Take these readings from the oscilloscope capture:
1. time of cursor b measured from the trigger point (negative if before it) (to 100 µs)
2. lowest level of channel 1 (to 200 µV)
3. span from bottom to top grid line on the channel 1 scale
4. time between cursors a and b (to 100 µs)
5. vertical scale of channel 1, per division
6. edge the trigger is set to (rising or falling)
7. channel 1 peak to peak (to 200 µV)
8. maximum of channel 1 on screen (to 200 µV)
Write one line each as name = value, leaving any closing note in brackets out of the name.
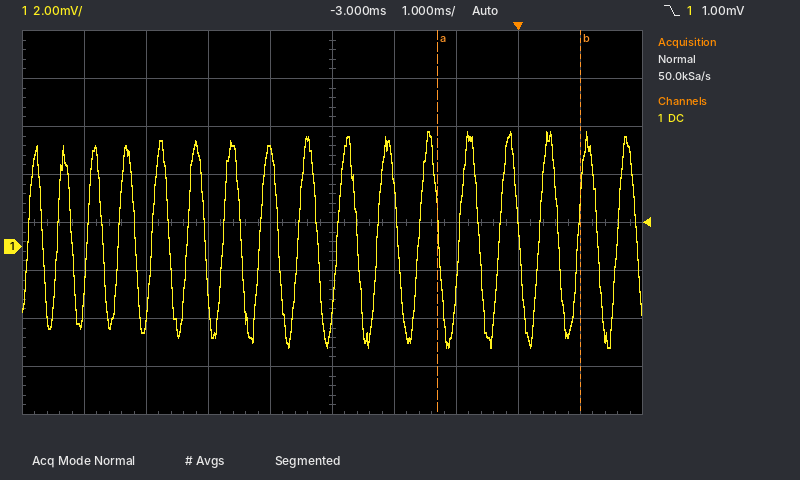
time of cursor b measured from the trigger point (negative if before it) = +1.0 ms
lowest level of channel 1 = -4.2 mV
span from bottom to top grid line on the channel 1 scale = 16 mV
time between cursors a and b = 2.3 ms
vertical scale of channel 1, per division = 2 mV
edge the trigger is set to = falling
channel 1 peak to peak = 9.0 mV
maximum of channel 1 on screen = 4.8 mV
